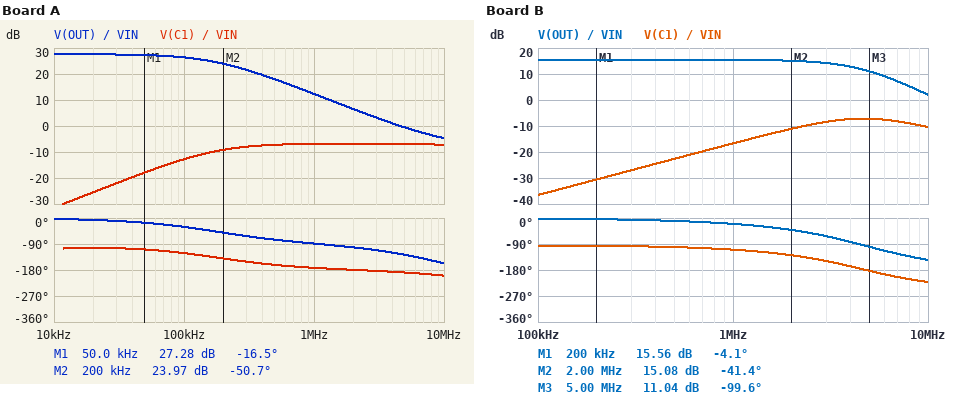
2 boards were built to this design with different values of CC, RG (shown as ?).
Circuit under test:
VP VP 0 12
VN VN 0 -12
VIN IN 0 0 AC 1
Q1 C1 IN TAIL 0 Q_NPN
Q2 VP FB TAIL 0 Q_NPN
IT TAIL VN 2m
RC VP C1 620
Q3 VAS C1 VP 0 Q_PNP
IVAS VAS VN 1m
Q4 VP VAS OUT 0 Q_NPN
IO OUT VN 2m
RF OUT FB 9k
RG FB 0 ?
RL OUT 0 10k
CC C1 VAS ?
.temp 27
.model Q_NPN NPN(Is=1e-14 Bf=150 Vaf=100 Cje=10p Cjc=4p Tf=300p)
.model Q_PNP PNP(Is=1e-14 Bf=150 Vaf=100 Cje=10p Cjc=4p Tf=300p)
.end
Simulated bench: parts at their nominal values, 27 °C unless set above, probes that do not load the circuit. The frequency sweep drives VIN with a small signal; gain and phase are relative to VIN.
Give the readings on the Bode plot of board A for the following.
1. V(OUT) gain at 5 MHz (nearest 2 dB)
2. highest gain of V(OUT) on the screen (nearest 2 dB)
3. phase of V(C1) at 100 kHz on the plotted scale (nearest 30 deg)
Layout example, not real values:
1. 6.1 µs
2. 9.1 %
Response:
1. 0 dB
2. 28 dB
3. -120 deg
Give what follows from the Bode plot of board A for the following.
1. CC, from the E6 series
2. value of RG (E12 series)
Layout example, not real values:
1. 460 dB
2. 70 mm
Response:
1. 680 pF
2. 390 Ω
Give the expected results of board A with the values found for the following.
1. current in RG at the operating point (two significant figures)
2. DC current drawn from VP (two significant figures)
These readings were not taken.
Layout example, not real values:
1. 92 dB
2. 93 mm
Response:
1. 9.1 µA
2. 5.0 mA
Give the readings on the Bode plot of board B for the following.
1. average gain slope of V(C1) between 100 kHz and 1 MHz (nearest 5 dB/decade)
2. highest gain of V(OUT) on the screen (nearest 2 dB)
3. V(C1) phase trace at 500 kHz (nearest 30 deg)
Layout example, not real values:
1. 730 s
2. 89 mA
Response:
1. 20 dB/decade
2. 16 dB
3. -90 deg
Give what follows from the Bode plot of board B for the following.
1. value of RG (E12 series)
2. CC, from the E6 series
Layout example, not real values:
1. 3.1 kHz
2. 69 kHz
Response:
1. 1.8 kΩ
2. 150 pF
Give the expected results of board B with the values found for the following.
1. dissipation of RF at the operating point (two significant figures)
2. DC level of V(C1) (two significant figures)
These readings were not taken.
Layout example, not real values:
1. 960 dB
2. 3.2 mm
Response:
1. 110 nW
2. 11 V
